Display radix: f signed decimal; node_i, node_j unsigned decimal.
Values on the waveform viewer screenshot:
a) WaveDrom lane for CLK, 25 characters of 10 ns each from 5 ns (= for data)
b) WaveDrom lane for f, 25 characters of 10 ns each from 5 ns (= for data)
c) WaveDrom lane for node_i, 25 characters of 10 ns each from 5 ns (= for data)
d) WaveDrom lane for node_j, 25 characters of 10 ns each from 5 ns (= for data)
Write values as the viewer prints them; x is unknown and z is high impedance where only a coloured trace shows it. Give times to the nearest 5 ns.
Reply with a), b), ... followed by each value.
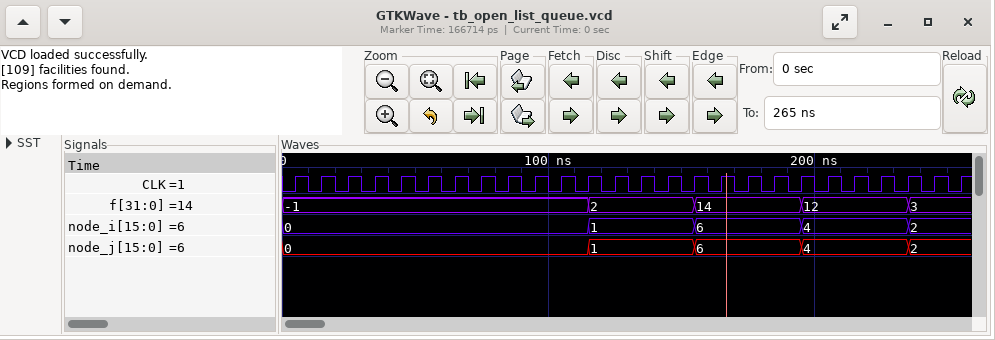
a) {name: 'CLK', wave: 'p........................'}
b) {name: 'f', wave: '=..........=...=...=...=.', data: '-1 2 14 12 3'}
c) {name: 'node_i', wave: '=..........=...=...=...=.', data: '0 1 6 4 2'}
d) {name: 'node_j', wave: '=..........=...=...=...=.', data: '0 1 6 4 2'}
